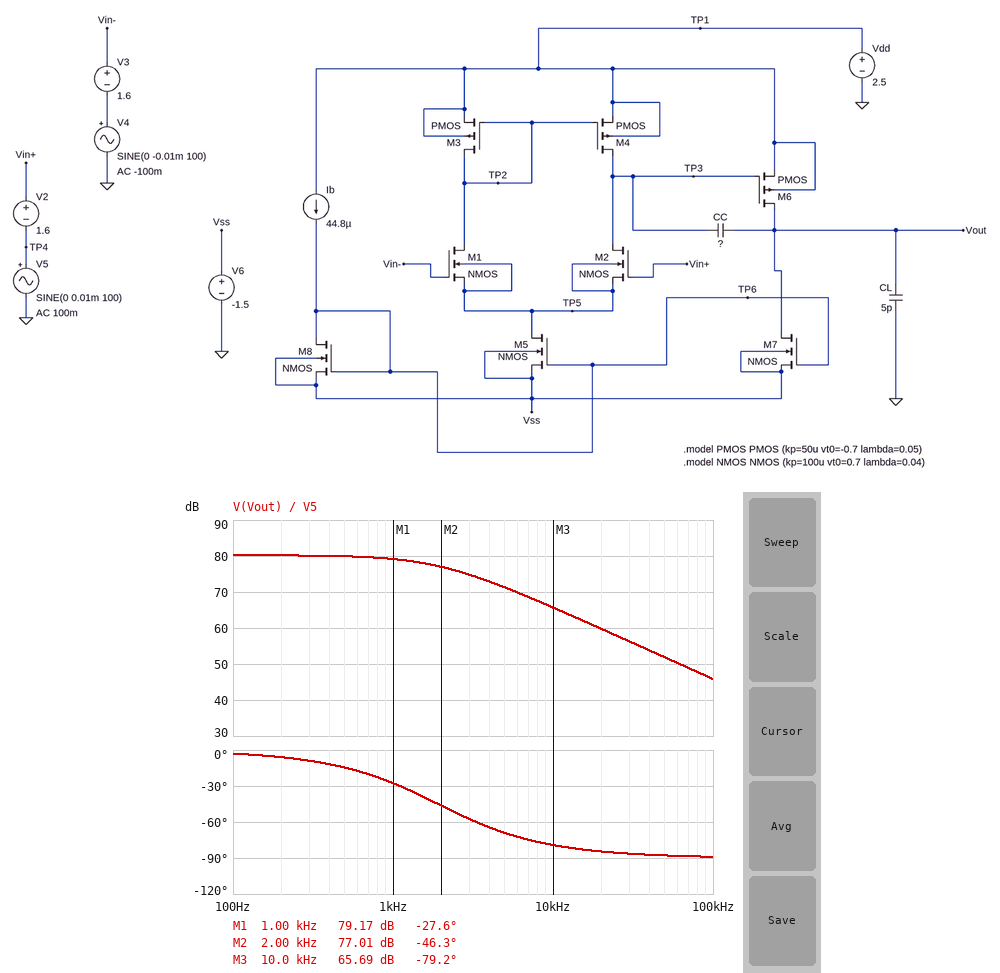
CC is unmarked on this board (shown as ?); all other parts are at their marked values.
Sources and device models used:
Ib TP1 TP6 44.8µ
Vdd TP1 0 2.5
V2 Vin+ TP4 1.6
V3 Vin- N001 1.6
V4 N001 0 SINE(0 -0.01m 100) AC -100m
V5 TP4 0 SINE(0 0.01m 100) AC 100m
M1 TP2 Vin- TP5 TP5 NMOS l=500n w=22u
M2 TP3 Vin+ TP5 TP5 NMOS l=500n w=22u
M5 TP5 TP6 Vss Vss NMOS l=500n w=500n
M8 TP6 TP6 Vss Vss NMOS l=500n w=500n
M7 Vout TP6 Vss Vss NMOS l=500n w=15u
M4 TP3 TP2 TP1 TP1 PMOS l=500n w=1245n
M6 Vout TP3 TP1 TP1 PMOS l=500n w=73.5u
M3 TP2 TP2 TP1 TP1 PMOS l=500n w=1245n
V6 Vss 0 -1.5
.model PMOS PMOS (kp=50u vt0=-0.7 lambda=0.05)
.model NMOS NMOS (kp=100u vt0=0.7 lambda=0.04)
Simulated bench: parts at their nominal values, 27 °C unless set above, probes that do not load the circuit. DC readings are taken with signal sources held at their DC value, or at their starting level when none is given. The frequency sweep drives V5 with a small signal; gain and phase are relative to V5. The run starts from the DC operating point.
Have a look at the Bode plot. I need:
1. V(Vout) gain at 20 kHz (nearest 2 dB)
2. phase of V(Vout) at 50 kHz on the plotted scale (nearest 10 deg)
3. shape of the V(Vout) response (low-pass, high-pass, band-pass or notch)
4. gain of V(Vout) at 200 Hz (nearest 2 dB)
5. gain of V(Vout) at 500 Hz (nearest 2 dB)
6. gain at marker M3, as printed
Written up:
60 dB
-90 deg
low-pass
80 dB
80 dB
65.69 dB
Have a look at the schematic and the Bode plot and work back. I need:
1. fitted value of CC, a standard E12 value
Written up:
3.9 pF
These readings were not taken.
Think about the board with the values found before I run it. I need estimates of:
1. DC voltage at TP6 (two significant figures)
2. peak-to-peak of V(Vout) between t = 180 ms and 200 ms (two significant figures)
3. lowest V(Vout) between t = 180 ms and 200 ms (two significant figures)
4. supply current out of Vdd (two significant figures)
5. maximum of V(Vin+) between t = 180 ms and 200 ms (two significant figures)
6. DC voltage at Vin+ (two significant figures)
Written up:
120 mV
370 mV
650 mV
1.5 mA
1.6 V
1.6 V
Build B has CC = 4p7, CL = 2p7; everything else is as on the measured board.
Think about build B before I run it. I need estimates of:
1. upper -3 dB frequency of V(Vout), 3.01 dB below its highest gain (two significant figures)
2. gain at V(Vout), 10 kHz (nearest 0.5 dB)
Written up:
1.6 kHz
64.0 dB
